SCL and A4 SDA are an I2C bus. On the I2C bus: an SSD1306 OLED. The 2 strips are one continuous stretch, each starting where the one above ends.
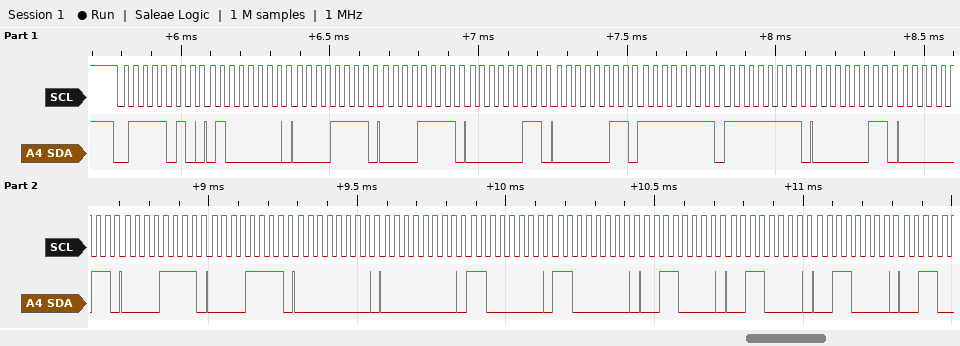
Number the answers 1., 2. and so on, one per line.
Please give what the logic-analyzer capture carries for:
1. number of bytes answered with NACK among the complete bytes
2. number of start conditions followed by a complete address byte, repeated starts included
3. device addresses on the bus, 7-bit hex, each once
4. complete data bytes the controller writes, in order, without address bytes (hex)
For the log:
1. 0
2. 1
3. 0x3D
4. 40 0F 0F 03 03 FF FF 03 03 0F 0F 00 00 C0 C0 30 30 30
